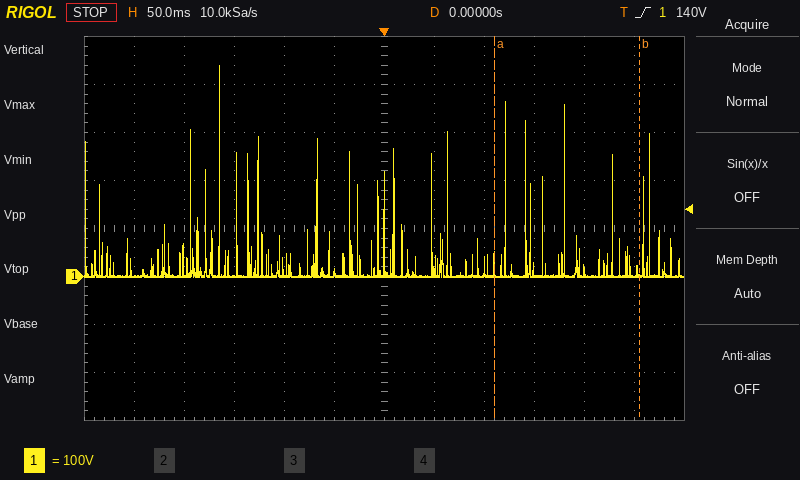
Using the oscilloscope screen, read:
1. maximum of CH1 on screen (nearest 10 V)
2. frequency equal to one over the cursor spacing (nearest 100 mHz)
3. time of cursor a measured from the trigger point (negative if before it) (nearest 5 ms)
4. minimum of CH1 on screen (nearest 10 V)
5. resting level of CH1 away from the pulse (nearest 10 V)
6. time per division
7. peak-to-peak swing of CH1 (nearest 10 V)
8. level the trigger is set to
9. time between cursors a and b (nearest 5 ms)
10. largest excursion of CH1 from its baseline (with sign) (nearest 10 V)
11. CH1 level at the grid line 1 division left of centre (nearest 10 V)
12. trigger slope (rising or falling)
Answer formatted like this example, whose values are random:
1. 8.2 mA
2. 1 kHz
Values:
1. 440 V
2. 6.9 Hz
3. +110 ms
4. 0 V
5. 0 V
6. 50 ms
7. 440 V
8. 140 V
9. 145 ms
10. +440 V
11. 10 V
12. rising
